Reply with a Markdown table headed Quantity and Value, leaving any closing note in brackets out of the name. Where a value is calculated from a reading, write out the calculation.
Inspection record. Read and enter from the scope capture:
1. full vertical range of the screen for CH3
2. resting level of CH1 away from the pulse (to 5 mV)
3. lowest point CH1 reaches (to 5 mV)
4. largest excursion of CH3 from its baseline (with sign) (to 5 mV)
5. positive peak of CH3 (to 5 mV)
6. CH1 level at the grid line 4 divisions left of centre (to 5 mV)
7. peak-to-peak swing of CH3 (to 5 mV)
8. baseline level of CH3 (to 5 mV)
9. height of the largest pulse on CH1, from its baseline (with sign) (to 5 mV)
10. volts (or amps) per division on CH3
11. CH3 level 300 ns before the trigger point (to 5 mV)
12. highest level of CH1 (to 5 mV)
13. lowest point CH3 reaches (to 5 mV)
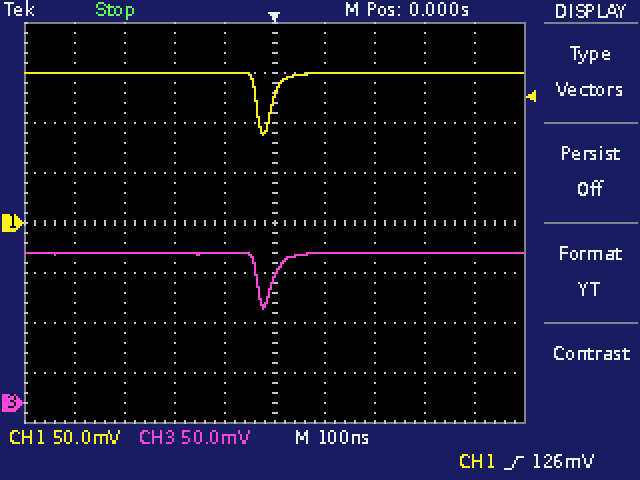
| Quantity | Value |
|---|---|
| full vertical range of the screen for CH3 | 400 mV |
| resting level of CH1 away from the pulse | 150 mV |
| lowest point CH1 reaches | 90 mV |
| largest excursion of CH3 from its baseline (with sign) | 95 mV − (150 mV) = -55 mV |
| positive peak of CH3 | 150 mV |
| CH1 level at the grid line 4 divisions left of centre | 150 mV |
| peak-to-peak swing of CH3 | 150 mV − (95 mV) = 55 mV |
| baseline level of CH3 | 150 mV |
| height of the largest pulse on CH1, from its baseline (with sign) | 90 mV − (150 mV) = -60 mV |
| volts (or amps) per division on CH3 | 50 mV |
| CH3 level 300 ns before the trigger point | 150 mV |
| highest level of CH1 | 150 mV |
| lowest point CH3 reaches | 95 mV |
